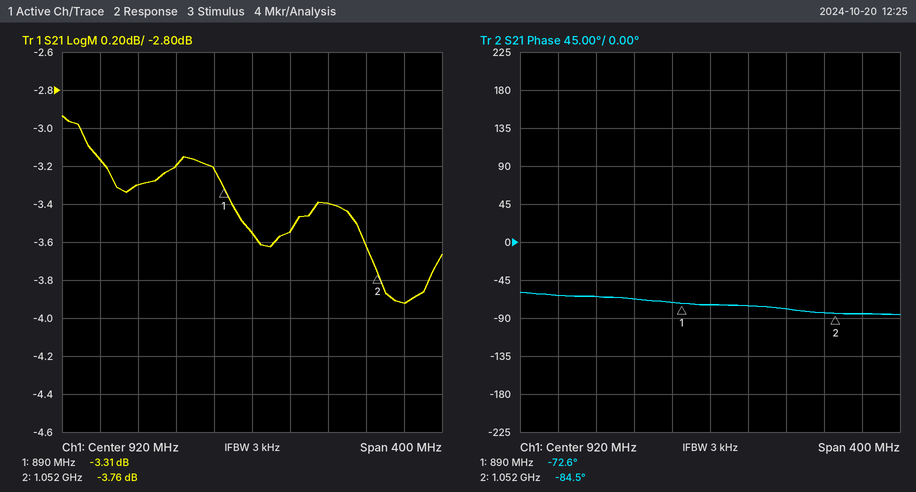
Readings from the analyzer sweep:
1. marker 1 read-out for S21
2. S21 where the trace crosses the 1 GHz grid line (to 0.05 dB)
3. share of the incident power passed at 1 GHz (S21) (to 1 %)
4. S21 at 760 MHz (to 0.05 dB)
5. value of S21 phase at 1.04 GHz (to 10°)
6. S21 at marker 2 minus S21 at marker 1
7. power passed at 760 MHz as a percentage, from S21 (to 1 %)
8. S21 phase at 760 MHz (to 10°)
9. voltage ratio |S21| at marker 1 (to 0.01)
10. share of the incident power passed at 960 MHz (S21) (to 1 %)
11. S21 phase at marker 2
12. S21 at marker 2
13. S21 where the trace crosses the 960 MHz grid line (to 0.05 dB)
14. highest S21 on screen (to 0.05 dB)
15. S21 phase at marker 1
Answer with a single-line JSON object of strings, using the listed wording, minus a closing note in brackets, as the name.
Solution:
{"marker 1 read-out for S21": "-3.31 dB", "S21 where the trace crosses the 1 GHz grid line": "-3.40 dB", "share of the incident power passed at 1 GHz (S21)": "46 %", "S21 at 760 MHz": "-3.15 dB", "value of S21 phase at 1.04 GHz": "-80°", "S21 at marker 2 minus S21 at marker 1": "-0.45 dB", "power passed at 760 MHz as a percentage, from S21": "48 %", "S21 phase at 760 MHz": "-60°", "voltage ratio |S21| at marker 1": "0.68", "share of the incident power passed at 960 MHz (S21)": "44 %", "S21 phase at marker 2": "-84.5°", "S21 at marker 2": "-3.76 dB", "S21 where the trace crosses the 960 MHz grid line": "-3.55 dB", "highest S21 on screen": "-2.95 dB", "S21 phase at marker 1": "-72.6°"}
